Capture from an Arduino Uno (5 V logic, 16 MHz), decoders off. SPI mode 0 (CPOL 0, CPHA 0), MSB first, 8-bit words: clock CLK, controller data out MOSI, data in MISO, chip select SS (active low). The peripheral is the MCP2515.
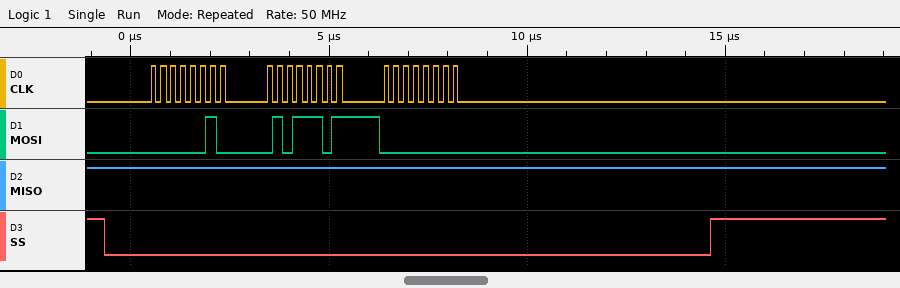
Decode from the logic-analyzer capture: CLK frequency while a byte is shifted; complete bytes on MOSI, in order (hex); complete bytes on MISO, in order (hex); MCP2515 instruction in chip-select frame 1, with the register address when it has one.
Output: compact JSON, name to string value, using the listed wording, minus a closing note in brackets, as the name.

{"CLK frequency while a byte is shifted": "4 MHz", "complete bytes on MOSI, in order": "02 5D 00", "complete bytes on MISO, in order": "FF FF FF", "MCP2515 instruction in chip-select frame 1, with the register address when it has one": "WRITE 0x5D"}
